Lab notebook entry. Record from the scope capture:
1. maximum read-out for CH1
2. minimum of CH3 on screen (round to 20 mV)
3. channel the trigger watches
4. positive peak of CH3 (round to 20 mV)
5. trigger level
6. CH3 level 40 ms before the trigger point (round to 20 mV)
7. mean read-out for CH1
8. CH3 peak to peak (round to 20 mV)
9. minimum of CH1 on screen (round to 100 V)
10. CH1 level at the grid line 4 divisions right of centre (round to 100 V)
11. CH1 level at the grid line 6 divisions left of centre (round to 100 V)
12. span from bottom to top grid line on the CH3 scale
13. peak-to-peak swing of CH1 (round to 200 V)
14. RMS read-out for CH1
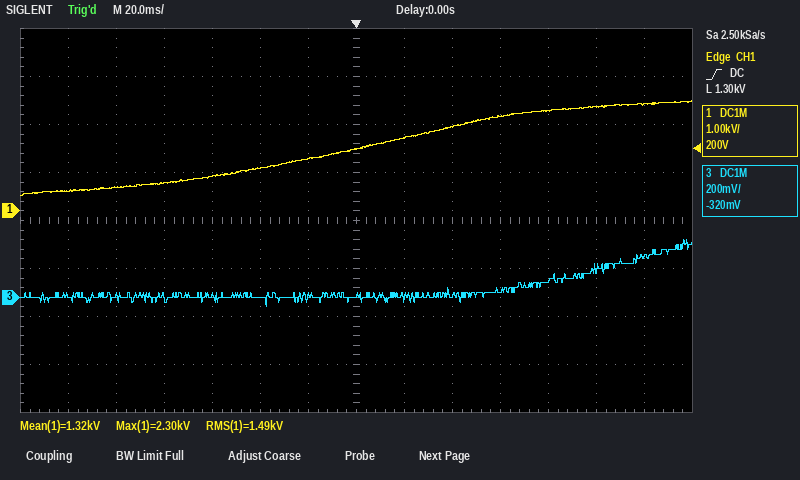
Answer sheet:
2.30 kV
-40 mV
CH1
240 mV
1.30 kV
0 mV
1.32 kV
280 mV
300 V
2.1 kV
400 V
1.6 V
2.0 kV
1.49 kV
